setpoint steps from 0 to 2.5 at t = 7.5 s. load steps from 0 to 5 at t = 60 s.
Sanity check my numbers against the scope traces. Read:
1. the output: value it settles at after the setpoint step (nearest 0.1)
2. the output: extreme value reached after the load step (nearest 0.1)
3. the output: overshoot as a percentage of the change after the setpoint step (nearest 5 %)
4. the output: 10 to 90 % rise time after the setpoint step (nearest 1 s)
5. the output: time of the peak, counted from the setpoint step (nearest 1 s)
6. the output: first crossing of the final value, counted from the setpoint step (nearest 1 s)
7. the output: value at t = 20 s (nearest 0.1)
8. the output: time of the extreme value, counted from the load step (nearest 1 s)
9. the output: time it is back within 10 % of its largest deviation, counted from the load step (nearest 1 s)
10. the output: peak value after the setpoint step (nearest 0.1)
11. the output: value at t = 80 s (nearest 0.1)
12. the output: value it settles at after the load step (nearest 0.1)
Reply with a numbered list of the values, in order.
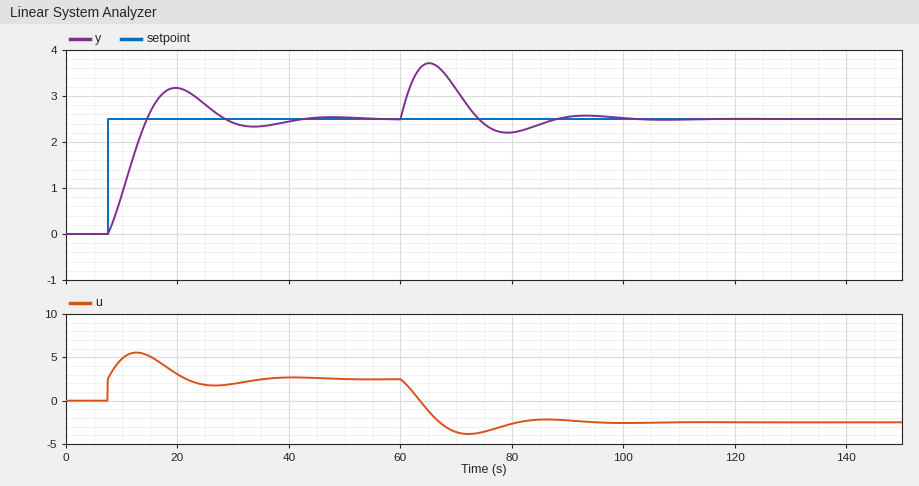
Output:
1. 2.5
2. 3.7
3. 25 %
4. 5 s
5. 12 s
6. 7 s
7. 3.2
8. 5 s
9. 25 s
10. 3.2
11. 2.2
12. 2.5
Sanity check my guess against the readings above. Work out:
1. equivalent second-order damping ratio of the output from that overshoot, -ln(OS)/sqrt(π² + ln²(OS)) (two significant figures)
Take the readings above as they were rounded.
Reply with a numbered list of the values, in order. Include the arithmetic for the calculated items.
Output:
1. ln(0.25) = -1.386; 1.386 / sqrt(9.870 + 1.922) = 0.40
